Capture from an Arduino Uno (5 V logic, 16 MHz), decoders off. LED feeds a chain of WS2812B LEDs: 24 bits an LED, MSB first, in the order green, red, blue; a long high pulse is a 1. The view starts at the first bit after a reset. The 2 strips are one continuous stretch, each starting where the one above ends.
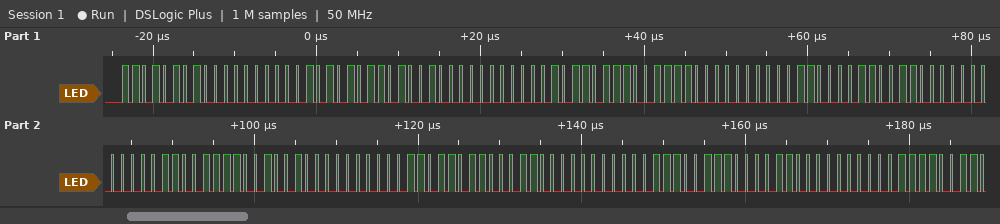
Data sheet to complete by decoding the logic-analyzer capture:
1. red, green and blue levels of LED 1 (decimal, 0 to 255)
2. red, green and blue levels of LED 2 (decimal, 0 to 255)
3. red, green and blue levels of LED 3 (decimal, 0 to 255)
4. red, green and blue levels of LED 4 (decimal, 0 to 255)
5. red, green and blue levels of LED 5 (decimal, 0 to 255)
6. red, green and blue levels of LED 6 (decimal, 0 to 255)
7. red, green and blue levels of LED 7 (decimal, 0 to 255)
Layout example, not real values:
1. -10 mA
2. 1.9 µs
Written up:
1. 0, 213, 42
2. 0, 210, 45
3. 0, 207, 48
4. 0, 204, 51
5. 0, 201, 54
6. 0, 198, 57
7. 0, 195, 60
